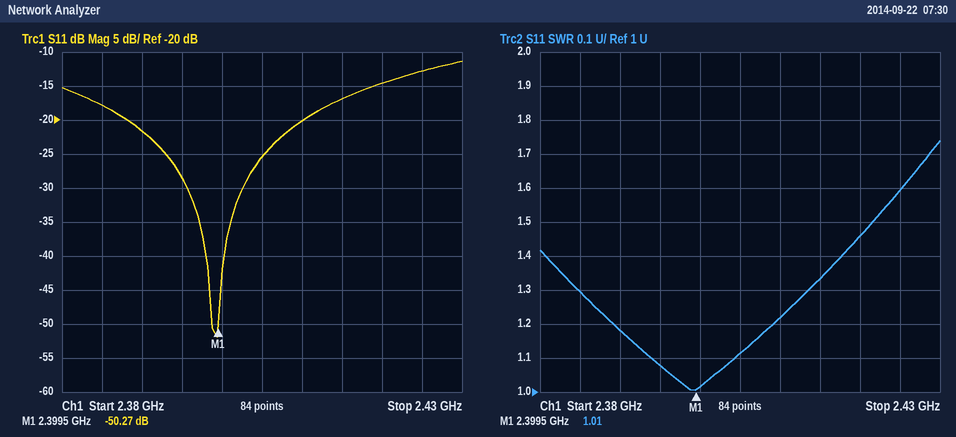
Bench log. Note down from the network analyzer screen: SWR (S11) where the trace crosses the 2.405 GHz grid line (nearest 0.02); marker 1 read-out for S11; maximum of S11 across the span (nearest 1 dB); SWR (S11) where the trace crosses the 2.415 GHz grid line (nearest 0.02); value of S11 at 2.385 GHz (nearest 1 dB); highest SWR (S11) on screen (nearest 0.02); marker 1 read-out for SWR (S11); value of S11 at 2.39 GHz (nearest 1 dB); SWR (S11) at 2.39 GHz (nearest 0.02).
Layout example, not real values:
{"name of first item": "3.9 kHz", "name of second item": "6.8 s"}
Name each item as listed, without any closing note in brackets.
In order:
{"SWR (S11) where the trace crosses the 2.405 GHz grid line": "1.12", "marker 1 read-out for S11": "-50.27 dB", "maximum of S11 across the span": "-11 dB", "SWR (S11) where the trace crosses the 2.415 GHz grid line": "1.34", "value of S11 at 2.385 GHz": "-18 dB", "highest SWR (S11) on screen": "1.74", "marker 1 read-out for SWR": "1.01", "value of S11 at 2.39 GHz": "-22 dB", "SWR (S11) at 2.39 GHz": "1.18"}
